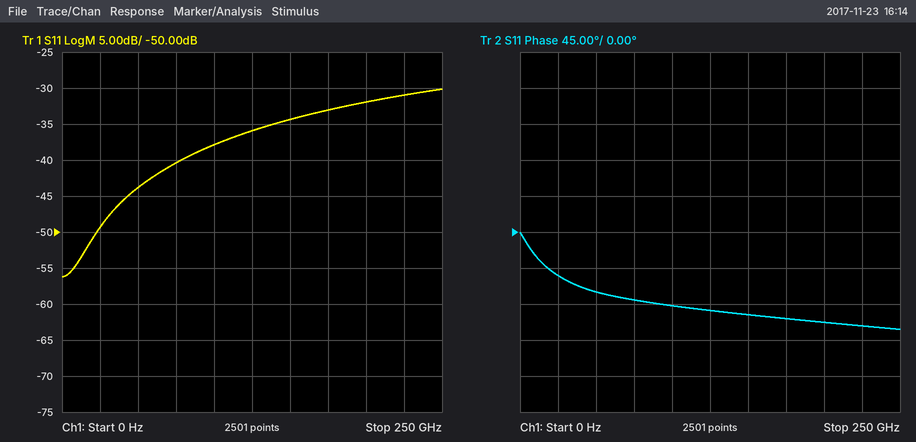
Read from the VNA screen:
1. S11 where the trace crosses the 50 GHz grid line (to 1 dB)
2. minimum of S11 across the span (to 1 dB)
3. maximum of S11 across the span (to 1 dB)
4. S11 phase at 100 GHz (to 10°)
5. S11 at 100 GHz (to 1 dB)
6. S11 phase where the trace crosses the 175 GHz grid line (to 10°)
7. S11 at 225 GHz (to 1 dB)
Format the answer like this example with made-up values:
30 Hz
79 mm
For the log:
-44 dB
-56 dB
-30 dB
-90°
-38 dB
-110°
-31 dB
